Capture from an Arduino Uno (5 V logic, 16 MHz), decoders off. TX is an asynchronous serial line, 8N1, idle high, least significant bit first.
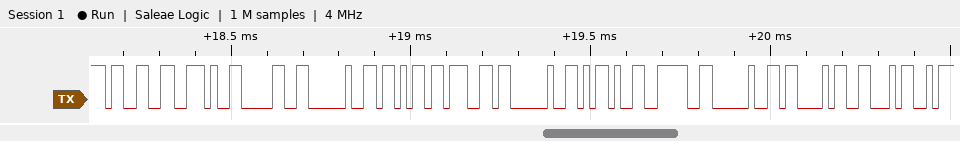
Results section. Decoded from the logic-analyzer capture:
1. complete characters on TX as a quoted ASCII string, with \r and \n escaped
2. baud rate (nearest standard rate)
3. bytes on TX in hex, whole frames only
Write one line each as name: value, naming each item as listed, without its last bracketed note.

complete characters on TX as a quoted ASCII string, with \r and \n escaped: "3.0 kg -> CF"
baud rate: 57600 baud
bytes on TX in hex, whole frames only: 0x33 0x2E 0x30 0x20 0x6B 0x67 0x20 0x2D 0x3E 0x20 0x43 0x46
